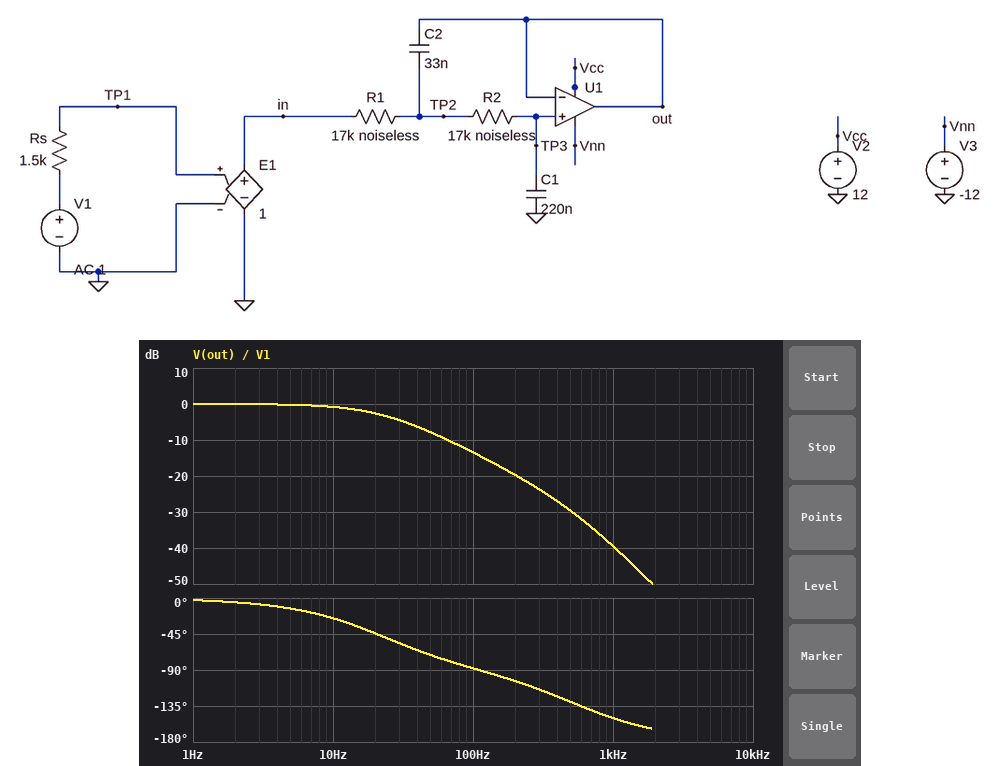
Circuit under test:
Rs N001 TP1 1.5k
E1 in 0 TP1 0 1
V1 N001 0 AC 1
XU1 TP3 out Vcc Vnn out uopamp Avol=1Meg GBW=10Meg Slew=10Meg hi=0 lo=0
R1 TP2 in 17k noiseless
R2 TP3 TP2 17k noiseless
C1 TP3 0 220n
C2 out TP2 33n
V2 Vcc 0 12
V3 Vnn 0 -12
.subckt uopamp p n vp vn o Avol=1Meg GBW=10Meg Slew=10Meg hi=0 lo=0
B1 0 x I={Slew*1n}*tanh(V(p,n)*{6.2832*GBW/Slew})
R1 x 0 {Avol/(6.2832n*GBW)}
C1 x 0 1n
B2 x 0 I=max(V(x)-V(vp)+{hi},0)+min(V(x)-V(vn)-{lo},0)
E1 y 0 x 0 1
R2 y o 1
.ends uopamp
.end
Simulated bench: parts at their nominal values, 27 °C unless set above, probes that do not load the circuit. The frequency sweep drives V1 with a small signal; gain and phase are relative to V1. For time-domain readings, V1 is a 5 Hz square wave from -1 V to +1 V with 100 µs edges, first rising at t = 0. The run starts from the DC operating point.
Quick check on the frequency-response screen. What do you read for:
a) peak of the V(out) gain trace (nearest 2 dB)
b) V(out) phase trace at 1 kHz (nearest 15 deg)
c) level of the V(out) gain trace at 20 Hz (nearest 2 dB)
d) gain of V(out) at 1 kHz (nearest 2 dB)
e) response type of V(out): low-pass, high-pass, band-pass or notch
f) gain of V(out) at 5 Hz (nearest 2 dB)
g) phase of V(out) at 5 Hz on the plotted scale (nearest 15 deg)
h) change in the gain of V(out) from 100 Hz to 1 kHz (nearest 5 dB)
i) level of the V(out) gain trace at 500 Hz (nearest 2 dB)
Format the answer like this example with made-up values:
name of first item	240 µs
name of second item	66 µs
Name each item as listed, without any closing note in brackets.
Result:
peak of the V(out) gain trace	0 dB
V(out) phase trace at 1 kHz	-150 deg
level of the V(out) gain trace at 20 Hz	-2 dB
gain of V(out) at 1 kHz	-40 dB
response type of V(out): low-pass, high-pass, band-pass or notch	low-pass
gain of V(out) at 5 Hz	0 dB
phase of V(out) at 5 Hz on the plotted scale	-15 deg
change in the gain of V(out) from 100 Hz to 1 kHz	-25 dB
level of the V(out) gain trace at 500 Hz	-30 dB
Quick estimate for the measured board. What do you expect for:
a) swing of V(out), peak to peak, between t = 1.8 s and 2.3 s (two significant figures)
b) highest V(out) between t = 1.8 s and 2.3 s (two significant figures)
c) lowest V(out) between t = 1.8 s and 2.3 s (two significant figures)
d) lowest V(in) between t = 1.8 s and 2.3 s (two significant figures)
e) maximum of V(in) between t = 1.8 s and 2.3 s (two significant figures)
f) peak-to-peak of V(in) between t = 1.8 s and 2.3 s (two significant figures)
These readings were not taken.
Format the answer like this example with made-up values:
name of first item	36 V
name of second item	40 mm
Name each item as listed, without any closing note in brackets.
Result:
swing of V(out), peak to peak, between t = 1.8 s and 2.3 s	2.0 V
highest V(out) between t = 1.8 s and 2.3 s	1.0 V
lowest V(out) between t = 1.8 s and 2.3 s	-1.0 V
lowest V(in) between t = 1.8 s and 2.3 s	-1.0 V
maximum of V(in) between t = 1.8 s and 2.3 s	1.0 V
peak-to-peak of V(in) between t = 1.8 s and 2.3 s	2.0 V
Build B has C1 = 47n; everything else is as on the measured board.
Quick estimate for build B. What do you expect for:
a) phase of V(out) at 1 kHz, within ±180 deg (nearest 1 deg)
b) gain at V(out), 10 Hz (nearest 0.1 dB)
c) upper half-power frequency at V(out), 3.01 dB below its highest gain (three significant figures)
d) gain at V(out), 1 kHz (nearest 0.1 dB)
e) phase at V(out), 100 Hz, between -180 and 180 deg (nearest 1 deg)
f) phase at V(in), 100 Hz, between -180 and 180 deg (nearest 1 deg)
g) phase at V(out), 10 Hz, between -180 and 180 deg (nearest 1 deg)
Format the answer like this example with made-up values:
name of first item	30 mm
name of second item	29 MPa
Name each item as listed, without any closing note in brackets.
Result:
phase of V(out) at 1 kHz, within ±180 deg	-149 deg
gain at V(out), 10 Hz	0 dB
upper half-power frequency at V(out), 3.01 dB below its highest gain	120 Hz
gain at V(out), 1 kHz	-25.8 dB
phase at V(out), 100 Hz, between -180 and 180 deg	-51 deg
phase at V(in), 100 Hz, between -180 and 180 deg	0 deg
phase at V(out), 10 Hz, between -180 and 180 deg	-6 deg
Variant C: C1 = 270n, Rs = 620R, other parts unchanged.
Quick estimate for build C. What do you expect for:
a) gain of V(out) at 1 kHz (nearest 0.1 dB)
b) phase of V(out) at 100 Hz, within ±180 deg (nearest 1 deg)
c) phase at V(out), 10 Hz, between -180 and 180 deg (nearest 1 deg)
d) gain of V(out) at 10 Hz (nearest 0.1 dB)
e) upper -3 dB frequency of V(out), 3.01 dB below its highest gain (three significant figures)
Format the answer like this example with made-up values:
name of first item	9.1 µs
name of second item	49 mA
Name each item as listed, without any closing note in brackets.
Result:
gain of V(out) at 1 kHz	-41.3 dB
phase of V(out) at 100 Hz, within ±180 deg	-90 deg
phase at V(out), 10 Hz, between -180 and 180 deg	-30 deg
gain of V(out) at 10 Hz	-1.2 dB
upper -3 dB frequency of V(out), 3.01 dB below its highest gain	17.9 Hz
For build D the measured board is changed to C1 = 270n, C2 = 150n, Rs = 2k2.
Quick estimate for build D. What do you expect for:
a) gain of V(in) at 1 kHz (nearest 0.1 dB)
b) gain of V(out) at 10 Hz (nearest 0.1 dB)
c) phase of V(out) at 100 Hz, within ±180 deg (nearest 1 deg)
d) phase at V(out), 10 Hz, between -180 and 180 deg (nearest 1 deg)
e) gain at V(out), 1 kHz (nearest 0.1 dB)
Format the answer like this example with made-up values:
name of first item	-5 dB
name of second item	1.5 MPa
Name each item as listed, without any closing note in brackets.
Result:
gain of V(in) at 1 kHz	0 dB
gain of V(out) at 10 Hz	-0.9 dB
phase of V(out) at 100 Hz, within ±180 deg	-122 deg
phase at V(out), 10 Hz, between -180 and 180 deg	-31 deg
gain at V(out), 1 kHz	-53.3 dB
